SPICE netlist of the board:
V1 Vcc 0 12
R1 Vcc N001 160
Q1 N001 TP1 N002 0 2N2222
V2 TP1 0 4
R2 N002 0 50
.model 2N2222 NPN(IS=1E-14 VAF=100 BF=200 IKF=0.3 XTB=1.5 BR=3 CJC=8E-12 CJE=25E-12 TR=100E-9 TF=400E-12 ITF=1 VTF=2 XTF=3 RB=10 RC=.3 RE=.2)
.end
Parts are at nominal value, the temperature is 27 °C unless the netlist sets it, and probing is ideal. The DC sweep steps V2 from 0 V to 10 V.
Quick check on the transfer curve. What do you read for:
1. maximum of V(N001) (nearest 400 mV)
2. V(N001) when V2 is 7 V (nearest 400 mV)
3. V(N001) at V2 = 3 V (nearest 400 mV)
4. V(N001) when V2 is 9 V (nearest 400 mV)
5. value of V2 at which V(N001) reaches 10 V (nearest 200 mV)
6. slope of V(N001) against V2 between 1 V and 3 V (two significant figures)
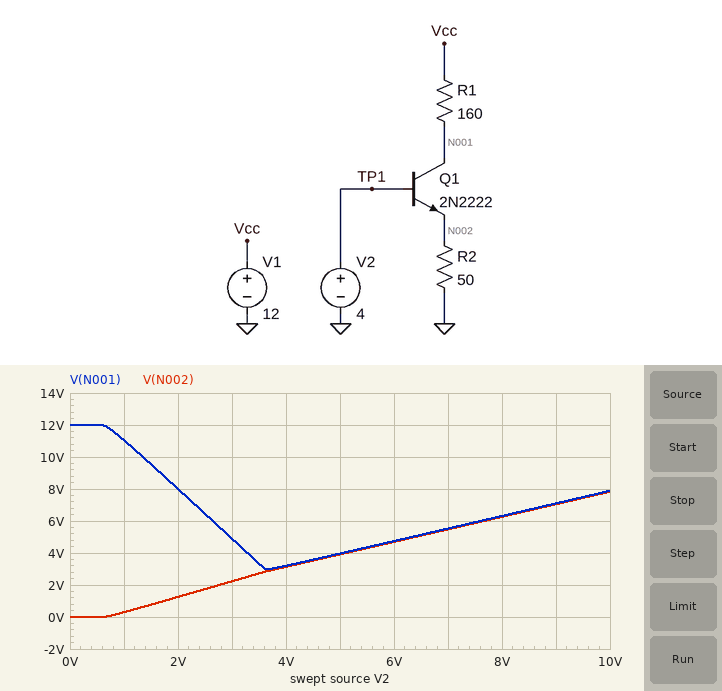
12.0 V
5.6 V
4.8 V
7.2 V
1.4 V
-3.1 V/V
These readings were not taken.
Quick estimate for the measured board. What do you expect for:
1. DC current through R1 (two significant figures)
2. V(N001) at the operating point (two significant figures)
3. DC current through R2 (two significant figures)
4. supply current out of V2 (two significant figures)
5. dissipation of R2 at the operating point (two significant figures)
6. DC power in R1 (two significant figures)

55 mA
3.2 V
63 mA
7.7 mA
200 mW
480 mW
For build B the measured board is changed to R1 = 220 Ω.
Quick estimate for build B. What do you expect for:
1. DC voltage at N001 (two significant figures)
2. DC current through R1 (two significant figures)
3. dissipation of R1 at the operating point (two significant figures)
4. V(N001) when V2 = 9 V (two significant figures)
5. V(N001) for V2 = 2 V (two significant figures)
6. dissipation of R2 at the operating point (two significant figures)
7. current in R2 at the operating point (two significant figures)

3.1 V
41 mA
360 mW
7.0 V
6.5 V
180 mW
60 mA
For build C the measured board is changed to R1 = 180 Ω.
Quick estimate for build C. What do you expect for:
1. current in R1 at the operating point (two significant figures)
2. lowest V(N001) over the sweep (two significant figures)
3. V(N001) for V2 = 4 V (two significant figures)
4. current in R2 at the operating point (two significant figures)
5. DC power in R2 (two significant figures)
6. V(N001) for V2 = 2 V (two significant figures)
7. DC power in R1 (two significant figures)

49 mA
2.7 V
3.1 V
62 mA
190 mW
7.5 V
440 mW
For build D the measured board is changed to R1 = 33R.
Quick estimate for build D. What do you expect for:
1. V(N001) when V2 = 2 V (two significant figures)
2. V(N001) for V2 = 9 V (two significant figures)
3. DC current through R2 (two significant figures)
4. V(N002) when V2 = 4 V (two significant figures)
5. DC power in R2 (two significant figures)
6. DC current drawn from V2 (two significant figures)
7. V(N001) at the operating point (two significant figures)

11 V
7.9 V
64 mA
3.2 V
210 mW
360 µA
9.9 V
